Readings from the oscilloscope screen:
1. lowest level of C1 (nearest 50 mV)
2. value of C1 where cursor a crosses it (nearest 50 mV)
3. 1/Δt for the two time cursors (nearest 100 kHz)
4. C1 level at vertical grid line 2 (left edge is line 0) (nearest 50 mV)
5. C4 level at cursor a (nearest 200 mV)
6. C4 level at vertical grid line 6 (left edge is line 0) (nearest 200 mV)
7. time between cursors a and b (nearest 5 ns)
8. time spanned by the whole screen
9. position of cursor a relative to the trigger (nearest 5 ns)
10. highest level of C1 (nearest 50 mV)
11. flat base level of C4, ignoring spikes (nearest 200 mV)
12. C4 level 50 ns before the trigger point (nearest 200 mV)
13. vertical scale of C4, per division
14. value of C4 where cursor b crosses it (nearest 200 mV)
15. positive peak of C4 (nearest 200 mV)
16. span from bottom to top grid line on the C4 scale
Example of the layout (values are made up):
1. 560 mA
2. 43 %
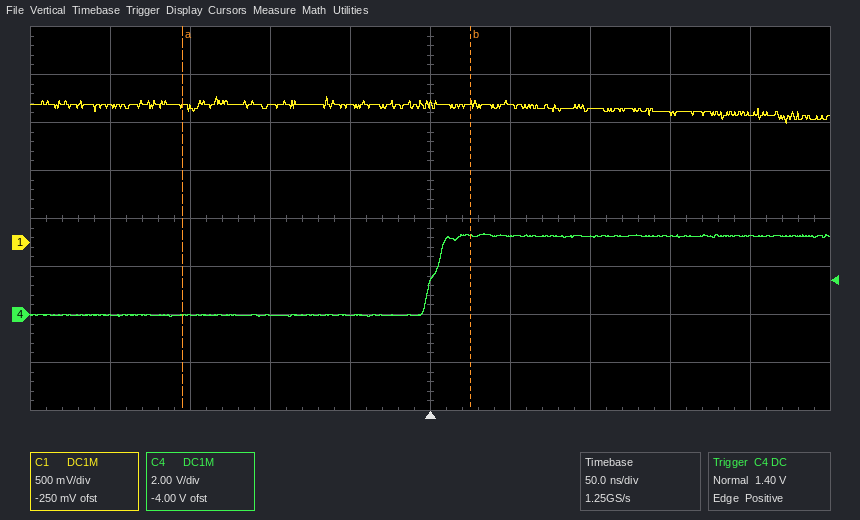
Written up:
1. 1.25 V
2. 1.40 V
3. 5.6 MHz
4. 1.40 V
5. 0.0 V
6. 3.2 V
7. 180 ns
8. 500 ns
9. -155 ns
10. 1.50 V
11. 0.0 V
12. 0.0 V
13. 2 V
14. 3.2 V
15. 3.4 V
16. 16 V
